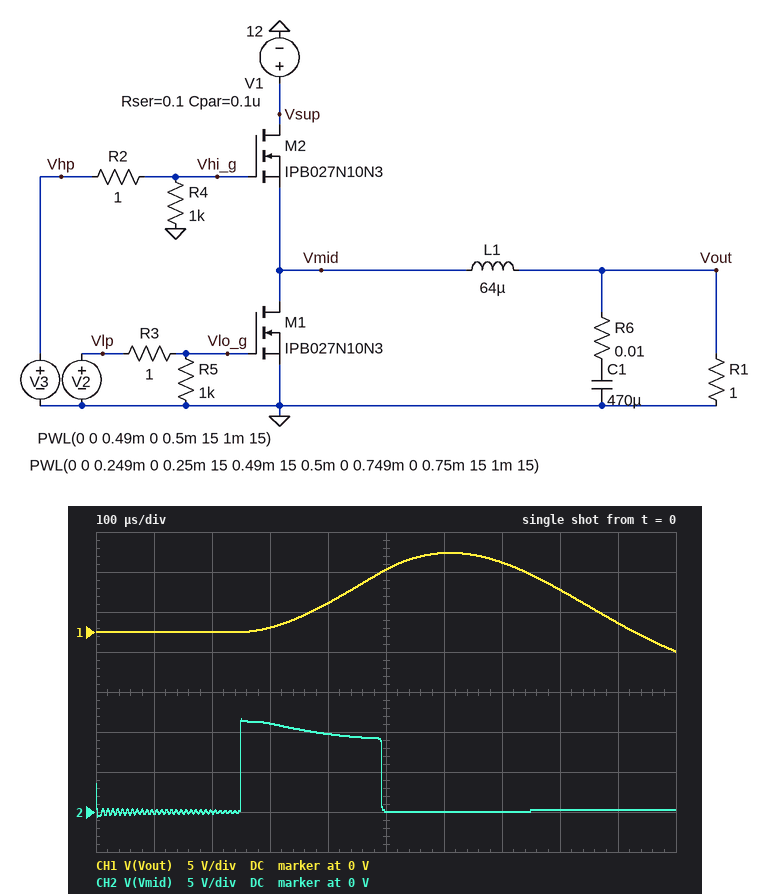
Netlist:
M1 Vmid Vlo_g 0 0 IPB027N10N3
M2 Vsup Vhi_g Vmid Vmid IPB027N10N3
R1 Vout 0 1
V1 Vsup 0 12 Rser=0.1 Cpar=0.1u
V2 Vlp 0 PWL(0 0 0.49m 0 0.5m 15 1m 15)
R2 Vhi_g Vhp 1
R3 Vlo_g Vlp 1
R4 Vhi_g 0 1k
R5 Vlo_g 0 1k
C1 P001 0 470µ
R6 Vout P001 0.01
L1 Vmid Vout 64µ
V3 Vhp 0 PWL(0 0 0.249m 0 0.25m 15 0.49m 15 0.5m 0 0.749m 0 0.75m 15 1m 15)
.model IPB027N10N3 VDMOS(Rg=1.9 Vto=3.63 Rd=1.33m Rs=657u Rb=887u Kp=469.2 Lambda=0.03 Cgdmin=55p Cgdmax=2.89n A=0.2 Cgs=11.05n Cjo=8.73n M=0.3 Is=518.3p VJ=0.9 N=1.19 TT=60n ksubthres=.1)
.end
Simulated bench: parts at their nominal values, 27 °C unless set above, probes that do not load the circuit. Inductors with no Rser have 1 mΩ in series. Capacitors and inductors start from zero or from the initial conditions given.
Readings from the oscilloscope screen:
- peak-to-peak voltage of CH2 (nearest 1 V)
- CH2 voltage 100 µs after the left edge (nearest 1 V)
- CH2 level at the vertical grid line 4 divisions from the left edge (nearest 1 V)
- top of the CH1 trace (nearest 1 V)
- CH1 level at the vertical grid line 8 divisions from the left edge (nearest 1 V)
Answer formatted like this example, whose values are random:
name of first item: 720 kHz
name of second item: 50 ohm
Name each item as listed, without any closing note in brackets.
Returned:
peak-to-peak voltage of CH2: 12 V
CH2 voltage 100 µs after the left edge: 0 V
CH2 level at the vertical grid line 4 divisions from the left edge: 10 V
top of the CH1 trace: 10 V
CH1 level at the vertical grid line 8 divisions from the left edge: 5 V
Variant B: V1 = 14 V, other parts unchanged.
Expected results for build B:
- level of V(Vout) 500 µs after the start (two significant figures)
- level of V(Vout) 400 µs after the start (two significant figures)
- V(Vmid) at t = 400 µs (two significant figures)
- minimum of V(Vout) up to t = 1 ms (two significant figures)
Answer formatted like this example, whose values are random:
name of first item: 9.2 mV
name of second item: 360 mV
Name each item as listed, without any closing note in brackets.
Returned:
level of V(Vout) 500 µs after the start: 8.3 V
level of V(Vout) 400 µs after the start: 3.7 V
V(Vmid) at t = 400 µs: 11 V
minimum of V(Vout) up to t = 1 ms: -2.5 V
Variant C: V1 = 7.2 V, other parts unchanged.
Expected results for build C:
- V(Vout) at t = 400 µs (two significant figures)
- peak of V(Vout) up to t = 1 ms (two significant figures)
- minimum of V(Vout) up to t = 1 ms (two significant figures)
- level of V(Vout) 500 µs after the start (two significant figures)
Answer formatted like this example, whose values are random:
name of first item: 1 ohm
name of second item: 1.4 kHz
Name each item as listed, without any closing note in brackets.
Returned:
V(Vout) at t = 400 µs: 2.2 V
peak of V(Vout) up to t = 1 ms: 6.0 V
minimum of V(Vout) up to t = 1 ms: -1.5 V
level of V(Vout) 500 µs after the start: 4.7 V
